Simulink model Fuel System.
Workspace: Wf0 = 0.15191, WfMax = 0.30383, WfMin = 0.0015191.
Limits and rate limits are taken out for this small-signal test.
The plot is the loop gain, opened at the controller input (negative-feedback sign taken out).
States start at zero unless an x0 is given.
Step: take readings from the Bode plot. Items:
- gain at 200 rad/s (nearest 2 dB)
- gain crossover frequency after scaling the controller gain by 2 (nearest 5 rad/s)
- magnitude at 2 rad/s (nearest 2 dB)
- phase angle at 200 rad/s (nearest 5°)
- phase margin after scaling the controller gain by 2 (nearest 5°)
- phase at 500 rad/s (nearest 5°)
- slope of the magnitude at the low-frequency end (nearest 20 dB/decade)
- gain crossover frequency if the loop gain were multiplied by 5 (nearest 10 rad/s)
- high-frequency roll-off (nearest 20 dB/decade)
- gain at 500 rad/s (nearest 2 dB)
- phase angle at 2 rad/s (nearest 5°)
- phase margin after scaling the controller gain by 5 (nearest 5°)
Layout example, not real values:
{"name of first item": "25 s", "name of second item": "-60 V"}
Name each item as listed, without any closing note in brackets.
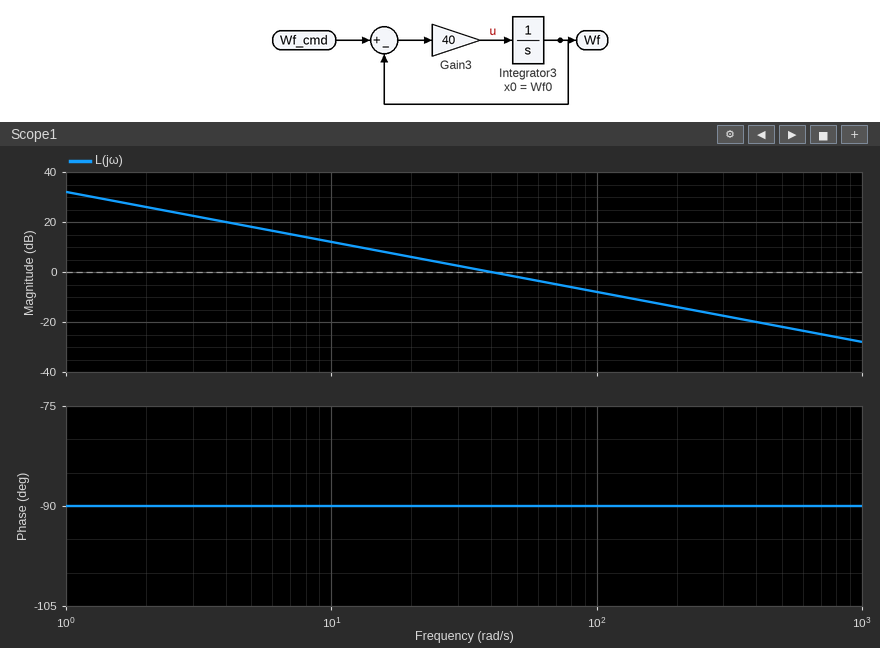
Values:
{"gain at 200 rad/s": "-14 dB", "gain crossover frequency after scaling the controller gain by 2": "80 rad/s", "magnitude at 2 rad/s": "26 dB", "phase angle at 200 rad/s": "-90°", "phase margin after scaling the controller gain by 2": "90°", "phase at 500 rad/s": "-90°", "slope of the magnitude at the low-frequency end": "-20 dB/decade", "gain crossover frequency if the loop gain were multiplied by 5": "200 rad/s", "high-frequency roll-off": "-20 dB/decade", "gain at 500 rad/s": "-22 dB", "phase angle at 2 rad/s": "-90°", "phase margin after scaling the controller gain by 5": "90°"}
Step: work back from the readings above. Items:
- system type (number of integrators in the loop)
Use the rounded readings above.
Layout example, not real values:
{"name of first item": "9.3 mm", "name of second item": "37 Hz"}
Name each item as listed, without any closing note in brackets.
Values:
{"system type": "1"}
